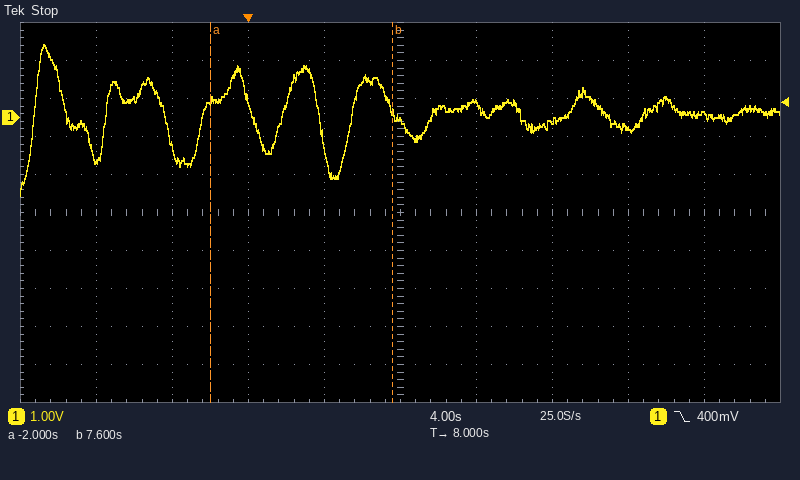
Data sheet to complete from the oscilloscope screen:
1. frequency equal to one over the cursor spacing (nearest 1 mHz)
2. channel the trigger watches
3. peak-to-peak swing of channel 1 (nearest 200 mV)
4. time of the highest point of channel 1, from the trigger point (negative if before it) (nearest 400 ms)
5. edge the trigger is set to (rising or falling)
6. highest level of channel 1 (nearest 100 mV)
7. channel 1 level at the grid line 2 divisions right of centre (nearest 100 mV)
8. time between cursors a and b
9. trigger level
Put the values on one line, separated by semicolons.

104 mHz; channel 1; 4.0 V; -10.8 s; falling; 1.9 V; -100 mV; 9.6 s; 400 mV
